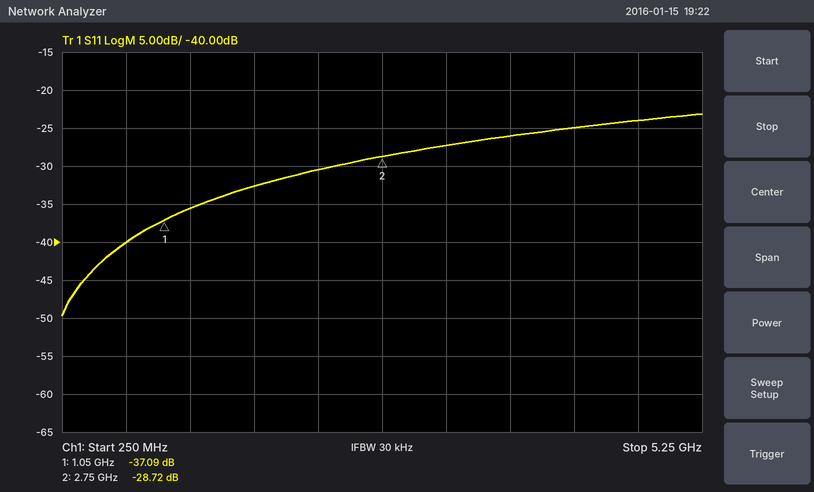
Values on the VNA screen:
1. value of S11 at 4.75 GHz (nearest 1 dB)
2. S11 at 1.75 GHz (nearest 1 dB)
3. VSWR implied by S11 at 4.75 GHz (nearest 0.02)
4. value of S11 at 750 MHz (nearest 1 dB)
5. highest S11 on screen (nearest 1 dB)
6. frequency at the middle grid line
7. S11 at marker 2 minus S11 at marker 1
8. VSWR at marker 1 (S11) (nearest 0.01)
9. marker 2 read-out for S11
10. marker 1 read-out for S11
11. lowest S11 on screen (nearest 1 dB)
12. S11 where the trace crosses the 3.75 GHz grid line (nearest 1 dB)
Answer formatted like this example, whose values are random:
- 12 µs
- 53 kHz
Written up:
- -24 dB
- -33 dB
- 1.14
- -40 dB
- -23 dB
- 2.75 GHz
- 8.37 dB
- 1.03
- -28.72 dB
- -37.09 dB
- -50 dB
- -26 dB
